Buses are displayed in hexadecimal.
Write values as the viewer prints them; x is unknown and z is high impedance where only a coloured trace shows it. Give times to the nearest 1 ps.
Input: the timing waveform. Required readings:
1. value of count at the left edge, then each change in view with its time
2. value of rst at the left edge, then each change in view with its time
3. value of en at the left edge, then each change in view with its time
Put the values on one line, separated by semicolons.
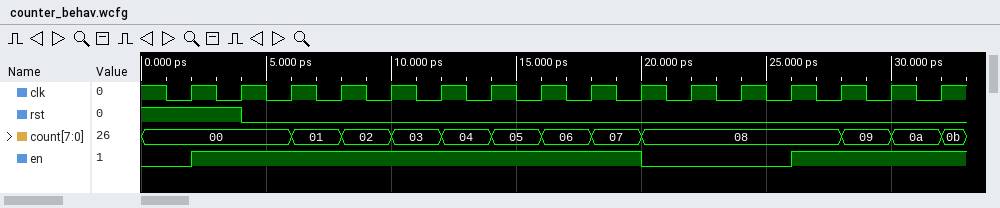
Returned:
00, 01 at 6 ps, 02 at 8 ps, 03 at 10 ps, 04 at 12 ps, 05 at 14 ps, 06 at 16 ps, 07 at 18 ps, 08 at 20 ps, 09 at 28 ps, 0a at 30 ps, 0b at 32 ps; 1, 0 at 4 ps; 0, 1 at 2 ps, 0 at 20 ps, 1 at 26 ps
